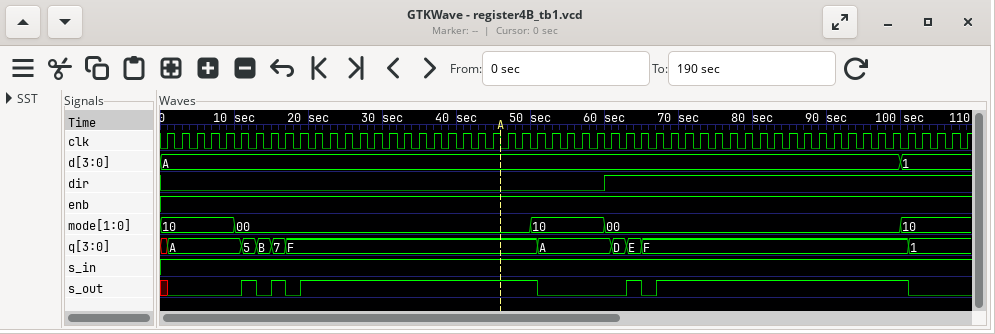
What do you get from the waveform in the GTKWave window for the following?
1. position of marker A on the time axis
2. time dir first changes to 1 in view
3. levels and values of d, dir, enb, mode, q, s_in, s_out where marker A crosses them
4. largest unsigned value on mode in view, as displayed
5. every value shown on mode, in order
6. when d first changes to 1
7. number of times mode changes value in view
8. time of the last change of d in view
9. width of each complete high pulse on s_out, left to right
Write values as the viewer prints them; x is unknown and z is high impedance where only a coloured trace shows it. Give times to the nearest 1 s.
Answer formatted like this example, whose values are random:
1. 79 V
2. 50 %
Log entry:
1. 46 s
2. 60 s
3. d=A, dir=0, enb=1, mode=00, q=F, s_in=1, s_out=1
4. 10
5. 10, 00, 10, 00, 10
6. 100 s
7. 4
8. 100 s
9. 2 s, 2 s, 32 s, 2 s, 34 s
